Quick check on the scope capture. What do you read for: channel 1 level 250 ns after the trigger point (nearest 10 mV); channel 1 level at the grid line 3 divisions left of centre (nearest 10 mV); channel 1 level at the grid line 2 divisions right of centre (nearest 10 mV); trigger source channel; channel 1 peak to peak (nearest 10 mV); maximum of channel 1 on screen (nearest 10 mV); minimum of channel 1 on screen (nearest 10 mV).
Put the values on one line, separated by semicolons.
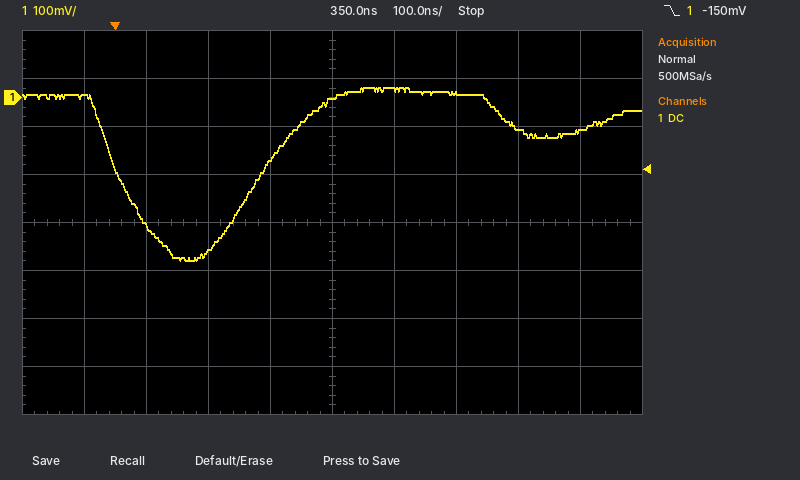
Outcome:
-130 mV; -270 mV; 10 mV; channel 1; 360 mV; 20 mV; -340 mV
